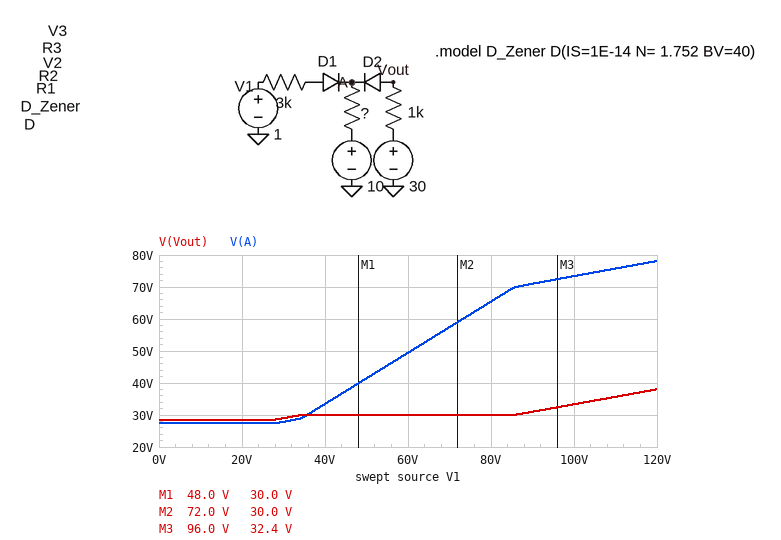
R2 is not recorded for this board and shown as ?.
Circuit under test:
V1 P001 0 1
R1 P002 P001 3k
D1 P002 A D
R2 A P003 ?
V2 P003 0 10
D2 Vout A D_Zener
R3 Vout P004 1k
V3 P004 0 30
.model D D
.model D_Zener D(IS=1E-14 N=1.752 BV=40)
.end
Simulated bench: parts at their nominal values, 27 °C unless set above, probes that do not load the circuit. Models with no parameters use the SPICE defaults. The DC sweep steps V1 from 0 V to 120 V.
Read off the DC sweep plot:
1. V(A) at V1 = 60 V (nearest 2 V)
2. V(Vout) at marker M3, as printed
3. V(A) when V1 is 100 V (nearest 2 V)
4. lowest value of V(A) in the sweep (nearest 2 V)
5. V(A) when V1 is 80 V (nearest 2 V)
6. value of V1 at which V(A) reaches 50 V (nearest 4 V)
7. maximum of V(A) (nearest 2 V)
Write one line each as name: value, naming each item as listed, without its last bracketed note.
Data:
V(A) at V1 = 60 V: 50 V
V(Vout) at marker M3, as printed: 32.4 V
V(A) when V1 is 100 V: 74 V
lowest value of V(A) in the sweep: 28 V
V(A) when V1 is 80 V: 66 V
value of V1 at which V(A) reaches 50 V: 60 V
maximum of V(A): 78 V
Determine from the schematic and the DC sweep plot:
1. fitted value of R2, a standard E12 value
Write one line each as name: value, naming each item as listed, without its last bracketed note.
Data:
fitted value of R2, a standard E12 value: 12 kΩ
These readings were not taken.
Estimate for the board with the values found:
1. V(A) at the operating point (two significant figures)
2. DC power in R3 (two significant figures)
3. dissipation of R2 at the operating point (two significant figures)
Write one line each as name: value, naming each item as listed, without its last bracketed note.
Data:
V(A) at the operating point: 27 V
DC power in R3: 2.1 mW
dissipation of R2 at the operating point: 25 mW
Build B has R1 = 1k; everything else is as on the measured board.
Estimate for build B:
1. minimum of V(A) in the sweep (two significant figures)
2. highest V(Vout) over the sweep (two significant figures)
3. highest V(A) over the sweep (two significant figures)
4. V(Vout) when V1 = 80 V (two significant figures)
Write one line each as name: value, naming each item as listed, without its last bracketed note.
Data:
minimum of V(A) in the sweep: 27 V
highest V(Vout) over the sweep: 51 V
highest V(A) over the sweep: 91 V
V(Vout) when V1 = 80 V: 32 V
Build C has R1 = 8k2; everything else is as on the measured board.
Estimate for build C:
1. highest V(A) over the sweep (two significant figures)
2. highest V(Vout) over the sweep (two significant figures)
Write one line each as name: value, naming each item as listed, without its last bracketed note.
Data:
highest V(A) over the sweep: 71 V
highest V(Vout) over the sweep: 31 V
